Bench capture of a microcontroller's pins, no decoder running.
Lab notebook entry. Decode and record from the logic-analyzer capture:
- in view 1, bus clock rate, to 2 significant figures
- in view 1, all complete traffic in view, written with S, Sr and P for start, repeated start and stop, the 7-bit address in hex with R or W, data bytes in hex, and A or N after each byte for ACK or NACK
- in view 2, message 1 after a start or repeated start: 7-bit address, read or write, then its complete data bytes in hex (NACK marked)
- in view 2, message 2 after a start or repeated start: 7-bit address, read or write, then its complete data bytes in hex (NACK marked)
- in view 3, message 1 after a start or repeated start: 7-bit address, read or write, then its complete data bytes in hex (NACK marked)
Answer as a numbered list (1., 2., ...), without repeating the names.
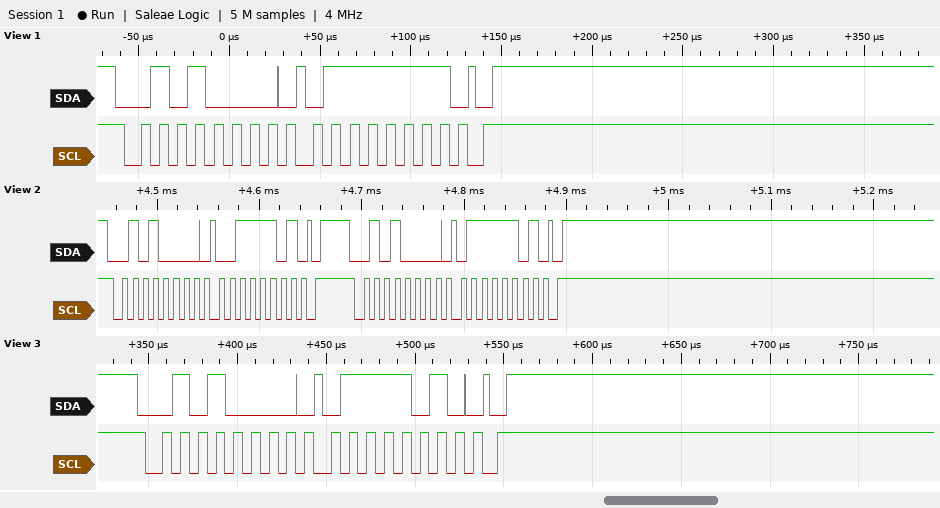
1. 100 kHz
2. S 28W A 7F A P
3. 0x28 write: 3D
4. 0x28 write: 7D
5. 0x28 write: 7A
